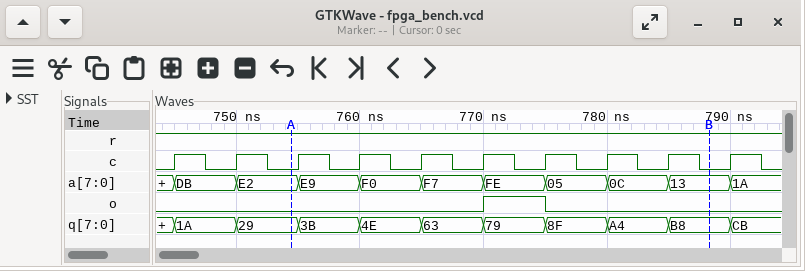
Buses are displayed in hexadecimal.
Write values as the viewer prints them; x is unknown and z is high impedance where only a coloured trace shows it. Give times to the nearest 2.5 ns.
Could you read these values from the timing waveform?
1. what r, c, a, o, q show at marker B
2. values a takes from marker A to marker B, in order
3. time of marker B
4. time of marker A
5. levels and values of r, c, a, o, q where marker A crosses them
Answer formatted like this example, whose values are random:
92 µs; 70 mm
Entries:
r=1, c=0, a=13, o=0, q=B8; E2, E9, F0, F7, FE, 05, 0C, 13; 787.5 ns; 755 ns; r=1, c=0, a=E2, o=0, q=29
